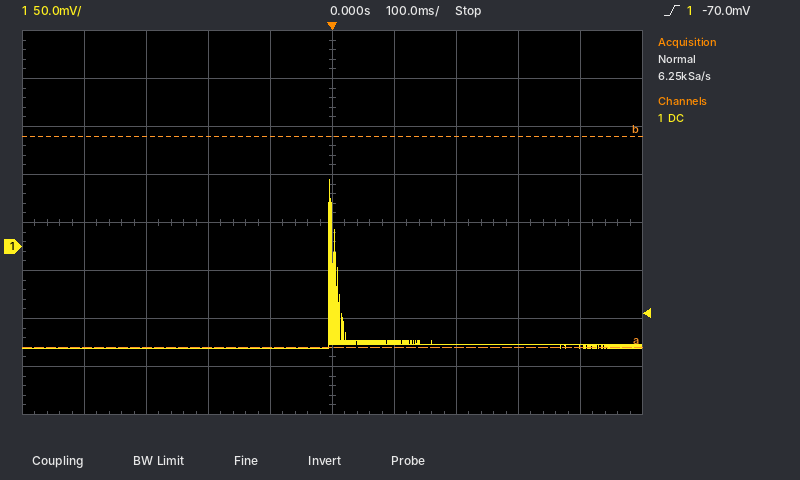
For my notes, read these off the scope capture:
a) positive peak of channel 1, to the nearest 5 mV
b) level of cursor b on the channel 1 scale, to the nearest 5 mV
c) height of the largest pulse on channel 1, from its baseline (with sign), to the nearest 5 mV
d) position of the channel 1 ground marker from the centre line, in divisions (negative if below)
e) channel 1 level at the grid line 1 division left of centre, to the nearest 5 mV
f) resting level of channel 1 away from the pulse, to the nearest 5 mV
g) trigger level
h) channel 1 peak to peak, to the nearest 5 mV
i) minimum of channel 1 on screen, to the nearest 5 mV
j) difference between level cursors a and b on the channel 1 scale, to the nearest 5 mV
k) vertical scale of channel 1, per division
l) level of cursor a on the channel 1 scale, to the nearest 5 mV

70 mV
115 mV
+175 mV
-0.5 div
-105 mV
-105 mV
-70.0 mV
175 mV
-105 mV
220 mV
50 mV
-105 mV
